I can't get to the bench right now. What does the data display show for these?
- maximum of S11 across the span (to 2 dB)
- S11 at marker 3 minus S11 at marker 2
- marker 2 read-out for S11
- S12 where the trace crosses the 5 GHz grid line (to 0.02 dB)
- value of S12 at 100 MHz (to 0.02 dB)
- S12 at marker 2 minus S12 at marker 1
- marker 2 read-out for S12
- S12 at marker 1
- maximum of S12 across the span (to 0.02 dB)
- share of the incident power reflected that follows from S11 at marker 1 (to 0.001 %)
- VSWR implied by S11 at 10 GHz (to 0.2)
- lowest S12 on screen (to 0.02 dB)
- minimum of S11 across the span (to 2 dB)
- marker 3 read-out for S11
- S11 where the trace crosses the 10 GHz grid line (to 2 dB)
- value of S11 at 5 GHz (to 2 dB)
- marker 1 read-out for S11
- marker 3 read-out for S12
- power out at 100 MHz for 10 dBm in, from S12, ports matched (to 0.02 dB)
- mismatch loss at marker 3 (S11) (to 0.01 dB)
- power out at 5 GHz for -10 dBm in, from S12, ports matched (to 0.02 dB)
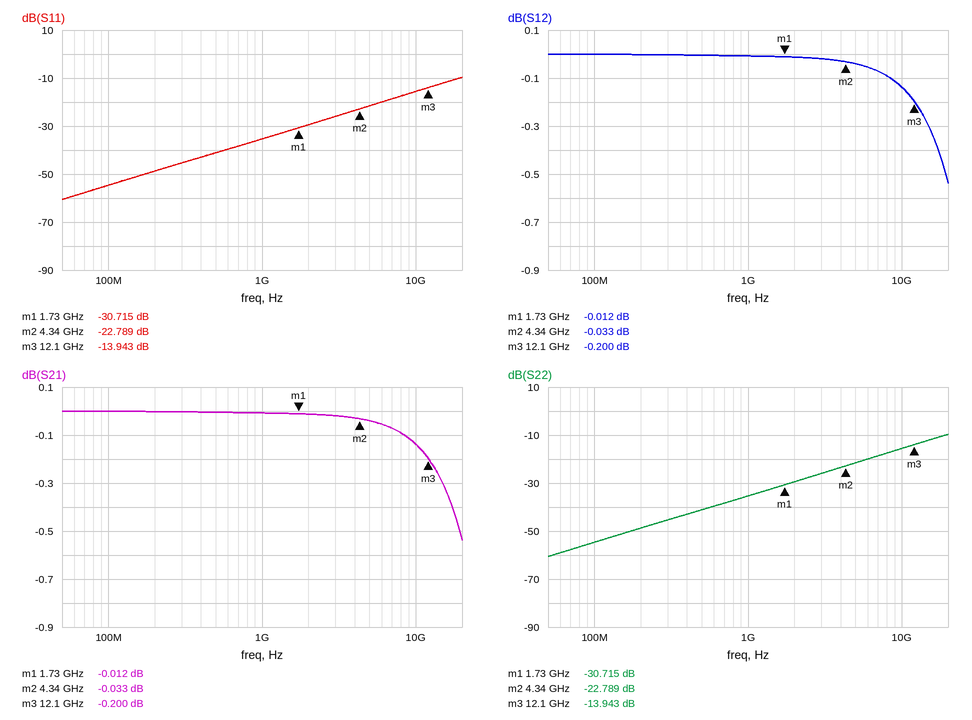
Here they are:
-10 dB
8.846 dB
-22.789 dB
-0.04 dB
0.00 dB
-0.021 dB
-0.033 dB
-0.012 dB
0.00 dB
0.085 %
1.4
-0.54 dB
-60 dB
-13.943 dB
-16 dB
-22 dB
-30.715 dB
-0.200 dB
10.00 dBm
0.18 dB
-10.04 dBm
